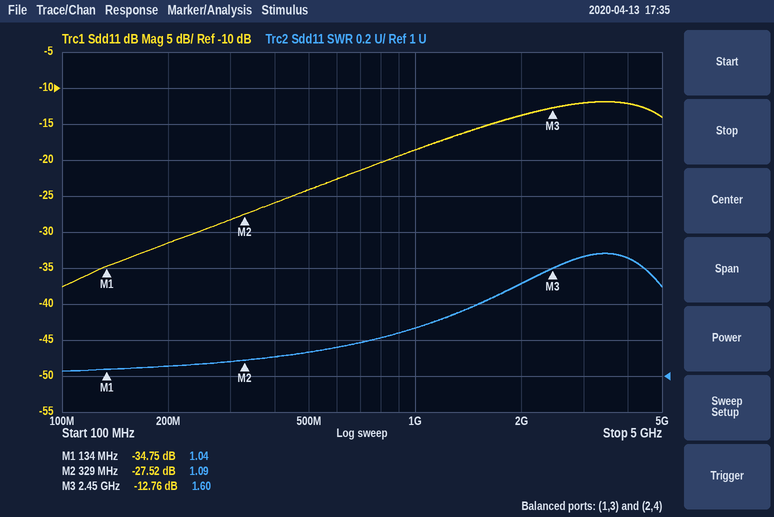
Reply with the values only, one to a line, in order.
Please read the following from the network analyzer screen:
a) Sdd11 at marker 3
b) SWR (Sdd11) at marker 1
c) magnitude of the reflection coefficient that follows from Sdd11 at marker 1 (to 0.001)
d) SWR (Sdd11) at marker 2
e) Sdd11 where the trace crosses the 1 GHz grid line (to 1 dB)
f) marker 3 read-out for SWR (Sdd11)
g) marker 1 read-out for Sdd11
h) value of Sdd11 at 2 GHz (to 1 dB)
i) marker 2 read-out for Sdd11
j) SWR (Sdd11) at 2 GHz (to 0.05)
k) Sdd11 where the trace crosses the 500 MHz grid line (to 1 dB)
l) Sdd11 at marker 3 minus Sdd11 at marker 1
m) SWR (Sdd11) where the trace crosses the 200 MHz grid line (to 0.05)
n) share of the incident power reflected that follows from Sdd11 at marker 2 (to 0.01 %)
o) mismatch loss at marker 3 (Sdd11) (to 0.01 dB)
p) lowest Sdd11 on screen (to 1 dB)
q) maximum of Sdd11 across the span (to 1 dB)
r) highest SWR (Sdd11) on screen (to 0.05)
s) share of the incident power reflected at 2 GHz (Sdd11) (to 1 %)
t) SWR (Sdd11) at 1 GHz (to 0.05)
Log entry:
-12.76 dB
1.04
0.018
1.09
-19 dB
1.60
-34.75 dB
-14 dB
-27.52 dB
1.50
-24 dB
21.99 dB
1.05
0.18 %
0.24 dB
-38 dB
-12 dB
1.70
4 %
1.25
